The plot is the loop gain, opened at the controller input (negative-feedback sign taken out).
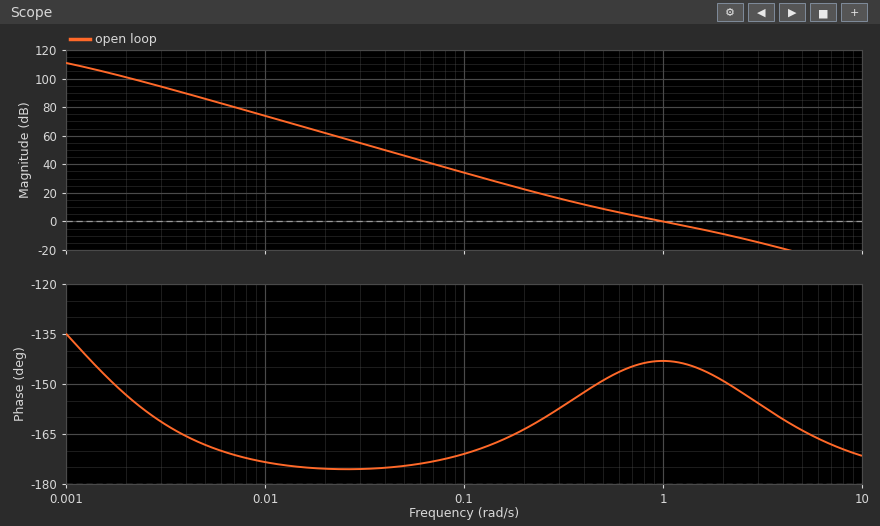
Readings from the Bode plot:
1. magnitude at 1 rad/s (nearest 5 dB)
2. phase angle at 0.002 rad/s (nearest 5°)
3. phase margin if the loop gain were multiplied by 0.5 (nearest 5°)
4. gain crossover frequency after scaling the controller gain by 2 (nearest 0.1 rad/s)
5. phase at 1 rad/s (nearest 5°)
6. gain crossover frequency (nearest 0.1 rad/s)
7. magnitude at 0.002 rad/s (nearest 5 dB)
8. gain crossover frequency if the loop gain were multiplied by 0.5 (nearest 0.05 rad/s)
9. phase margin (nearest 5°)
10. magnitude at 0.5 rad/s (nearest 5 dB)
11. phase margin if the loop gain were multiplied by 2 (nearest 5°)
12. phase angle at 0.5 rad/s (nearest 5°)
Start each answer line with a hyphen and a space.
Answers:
- 0 dB
- -155°
- 35°
- 1.6 rad/s
- -145°
- 1.0 rad/s
- 100 dB
- 0.60 rad/s
- 35°
- 10 dB
- 35°
- -150°
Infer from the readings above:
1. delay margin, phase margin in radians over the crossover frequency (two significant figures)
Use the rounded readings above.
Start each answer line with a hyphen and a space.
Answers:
- 0.61 s
